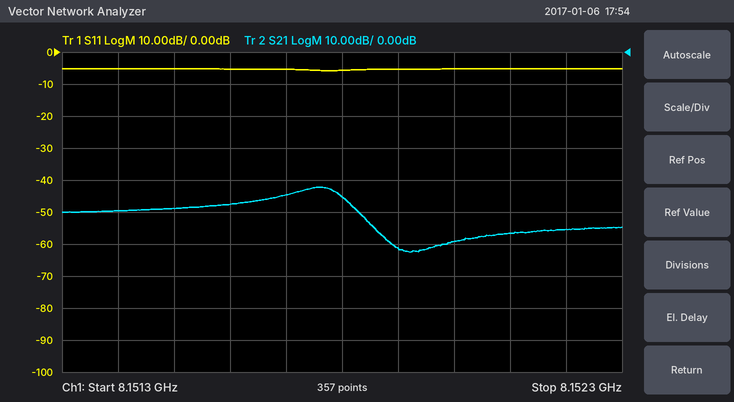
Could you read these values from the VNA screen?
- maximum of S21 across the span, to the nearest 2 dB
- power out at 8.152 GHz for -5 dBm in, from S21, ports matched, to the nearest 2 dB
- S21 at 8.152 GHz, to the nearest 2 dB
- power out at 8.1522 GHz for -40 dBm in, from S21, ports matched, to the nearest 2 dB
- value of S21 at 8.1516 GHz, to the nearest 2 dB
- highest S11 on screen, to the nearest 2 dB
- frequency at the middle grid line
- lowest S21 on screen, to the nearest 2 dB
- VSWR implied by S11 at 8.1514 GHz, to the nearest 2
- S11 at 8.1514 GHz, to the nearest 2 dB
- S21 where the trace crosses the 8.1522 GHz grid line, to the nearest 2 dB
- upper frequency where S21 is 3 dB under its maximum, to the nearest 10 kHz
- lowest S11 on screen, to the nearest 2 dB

-42 dB
-64 dBm
-60 dB
-96 dBm
-48 dB
-6 dB
8.1518 GHz
-62 dB
4
-6 dB
-56 dB
8.15180 GHz
-6 dB
